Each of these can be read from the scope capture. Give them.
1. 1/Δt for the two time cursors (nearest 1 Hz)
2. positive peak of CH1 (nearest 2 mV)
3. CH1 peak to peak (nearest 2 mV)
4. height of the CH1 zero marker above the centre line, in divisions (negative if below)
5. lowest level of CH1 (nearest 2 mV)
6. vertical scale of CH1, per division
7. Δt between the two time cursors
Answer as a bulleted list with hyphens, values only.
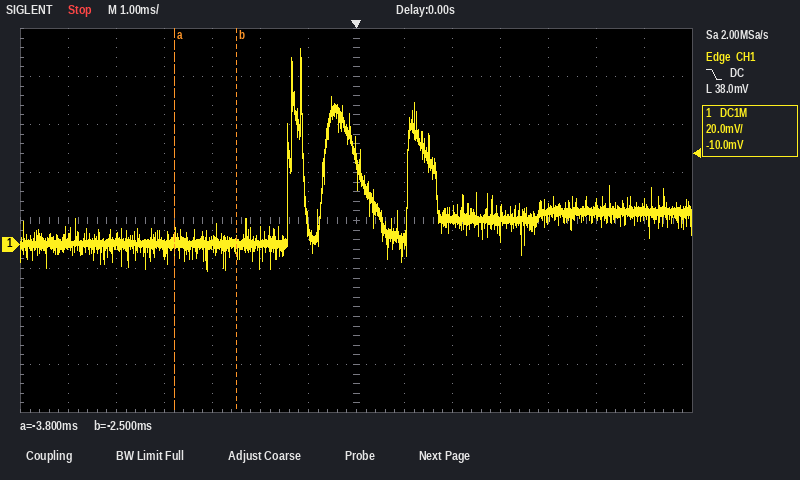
- 769 Hz
- 82 mV
- 92 mV
- -0.5 div
- -10 mV
- 20 mV
- 1.3 ms
